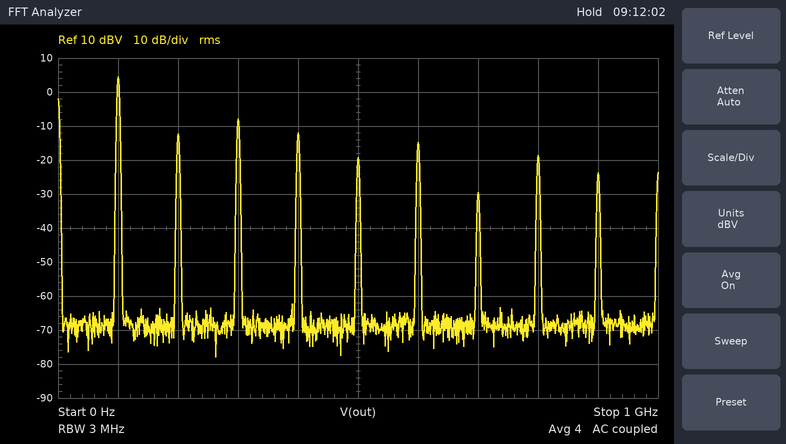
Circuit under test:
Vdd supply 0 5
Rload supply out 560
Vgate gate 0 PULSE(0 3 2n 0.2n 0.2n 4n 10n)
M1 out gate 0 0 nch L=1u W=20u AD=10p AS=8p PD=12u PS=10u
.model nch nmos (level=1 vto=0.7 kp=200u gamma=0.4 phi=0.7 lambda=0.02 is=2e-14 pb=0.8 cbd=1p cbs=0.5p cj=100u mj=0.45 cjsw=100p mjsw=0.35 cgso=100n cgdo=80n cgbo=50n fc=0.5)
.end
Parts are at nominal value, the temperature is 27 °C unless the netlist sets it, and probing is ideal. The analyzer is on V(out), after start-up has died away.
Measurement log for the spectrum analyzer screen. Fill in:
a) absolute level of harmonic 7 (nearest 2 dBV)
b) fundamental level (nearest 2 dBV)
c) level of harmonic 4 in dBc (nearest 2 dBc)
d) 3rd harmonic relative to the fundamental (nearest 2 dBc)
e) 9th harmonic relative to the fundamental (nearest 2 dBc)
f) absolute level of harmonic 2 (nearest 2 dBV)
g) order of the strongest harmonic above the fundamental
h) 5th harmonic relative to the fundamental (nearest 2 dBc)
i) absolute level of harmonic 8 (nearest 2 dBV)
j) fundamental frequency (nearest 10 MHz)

-30 dBV
4 dBV
-16 dBc
-12 dBc
-28 dBc
-12 dBV
3
-24 dBc
-18 dBV
100 MHz
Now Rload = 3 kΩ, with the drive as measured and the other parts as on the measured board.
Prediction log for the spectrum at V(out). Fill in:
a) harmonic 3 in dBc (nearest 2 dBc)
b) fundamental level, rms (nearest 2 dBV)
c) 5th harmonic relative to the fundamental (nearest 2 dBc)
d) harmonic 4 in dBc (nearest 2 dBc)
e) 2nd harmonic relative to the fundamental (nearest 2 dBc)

-10 dBc
0 dBV
-16 dBc
-14 dBc
-12 dBc
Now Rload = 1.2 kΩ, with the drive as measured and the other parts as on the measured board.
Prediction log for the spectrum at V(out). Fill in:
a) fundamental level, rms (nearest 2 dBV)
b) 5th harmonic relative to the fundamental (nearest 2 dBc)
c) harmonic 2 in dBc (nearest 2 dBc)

4 dBV
-20 dBc
-16 dBc
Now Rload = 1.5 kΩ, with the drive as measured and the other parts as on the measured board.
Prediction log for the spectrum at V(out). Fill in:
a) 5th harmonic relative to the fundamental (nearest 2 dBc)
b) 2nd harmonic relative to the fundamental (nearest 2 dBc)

-20 dBc
-14 dBc
